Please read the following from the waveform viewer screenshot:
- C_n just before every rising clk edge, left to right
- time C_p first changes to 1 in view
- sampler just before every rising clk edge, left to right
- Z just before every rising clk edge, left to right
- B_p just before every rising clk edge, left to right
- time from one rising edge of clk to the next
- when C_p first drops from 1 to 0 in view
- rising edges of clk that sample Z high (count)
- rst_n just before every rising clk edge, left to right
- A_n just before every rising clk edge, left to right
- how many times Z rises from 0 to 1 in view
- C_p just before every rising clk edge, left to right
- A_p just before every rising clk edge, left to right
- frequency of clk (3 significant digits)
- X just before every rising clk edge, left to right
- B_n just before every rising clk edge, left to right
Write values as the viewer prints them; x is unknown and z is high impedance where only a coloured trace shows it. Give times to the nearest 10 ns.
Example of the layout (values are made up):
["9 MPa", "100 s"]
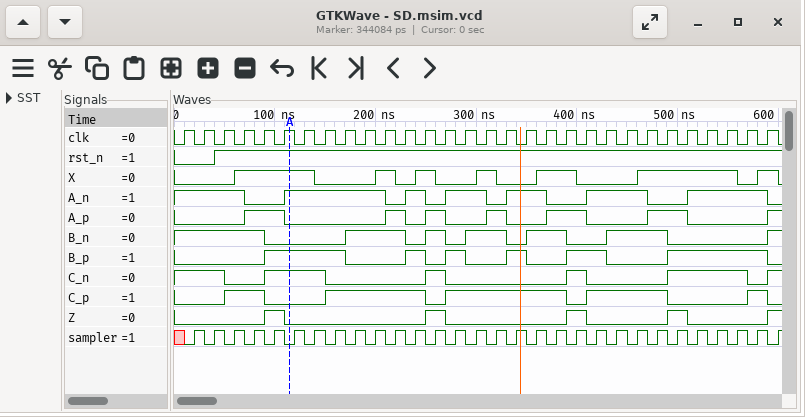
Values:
["1 1 1 0 0 1 1 1 0 0 0 0 0 1 0 0 0 0 0 0 1 0 0 0 0 1 1 1 1 0", "50 ns", "x 1 1 1 1 1 1 1 1 1 1 1 1 1 1 1 1 1 1 1 1 1 1 1 1 1 1 1 1 1", "0 0 0 0 0 1 0 0 0 0 0 0 0 1 0 0 0 0 0 0 1 0 0 0 0 1 0 0 0 0", "0 0 0 0 0 1 1 1 1 0 0 0 1 0 1 0 0 1 0 0 1 1 0 0 0 1 1 1 1 1", "20 ns", "90 ns", "4", "0 0 1 1 1 1 1 1 1 1 1 1 1 1 1 1 1 1 1 1 1 1 1 1 1 1 1 1 1 1", "1 1 1 1 0 0 1 1 1 1 1 0 1 0 1 1 0 1 1 0 0 1 1 1 0 0 1 1 1 1", "5", "0 0 0 1 1 0 0 0 1 1 1 1 1 0 1 1 1 1 1 1 0 1 1 1 1 0 0 0 0 1", "0 0 0 0 1 1 0 0 0 0 0 1 0 1 0 0 1 0 0 1 1 0 0 0 1 1 0 0 0 0", "50.0 MHz", "0 0 0 1 1 1 1 0 0 0 1 0 1 0 0 1 0 0 1 1 0 0 0 1 1 1 1 1 0 1", "1 1 1 1 1 0 0 0 0 1 1 1 0 1 0 1 1 0 1 1 0 0 1 1 1 0 0 0 0 0"]
